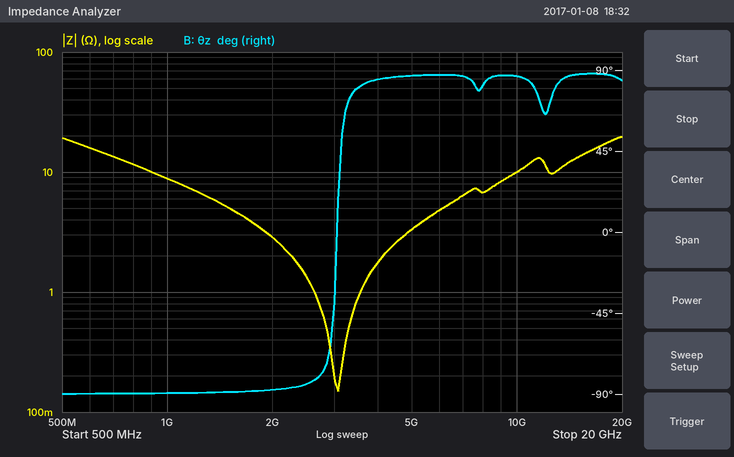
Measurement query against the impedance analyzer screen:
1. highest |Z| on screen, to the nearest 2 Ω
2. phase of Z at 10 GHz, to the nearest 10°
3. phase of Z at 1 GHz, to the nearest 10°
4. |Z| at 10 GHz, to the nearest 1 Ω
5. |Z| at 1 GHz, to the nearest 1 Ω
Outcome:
20 Ω
90°
-90°
10 Ω
9 Ω
